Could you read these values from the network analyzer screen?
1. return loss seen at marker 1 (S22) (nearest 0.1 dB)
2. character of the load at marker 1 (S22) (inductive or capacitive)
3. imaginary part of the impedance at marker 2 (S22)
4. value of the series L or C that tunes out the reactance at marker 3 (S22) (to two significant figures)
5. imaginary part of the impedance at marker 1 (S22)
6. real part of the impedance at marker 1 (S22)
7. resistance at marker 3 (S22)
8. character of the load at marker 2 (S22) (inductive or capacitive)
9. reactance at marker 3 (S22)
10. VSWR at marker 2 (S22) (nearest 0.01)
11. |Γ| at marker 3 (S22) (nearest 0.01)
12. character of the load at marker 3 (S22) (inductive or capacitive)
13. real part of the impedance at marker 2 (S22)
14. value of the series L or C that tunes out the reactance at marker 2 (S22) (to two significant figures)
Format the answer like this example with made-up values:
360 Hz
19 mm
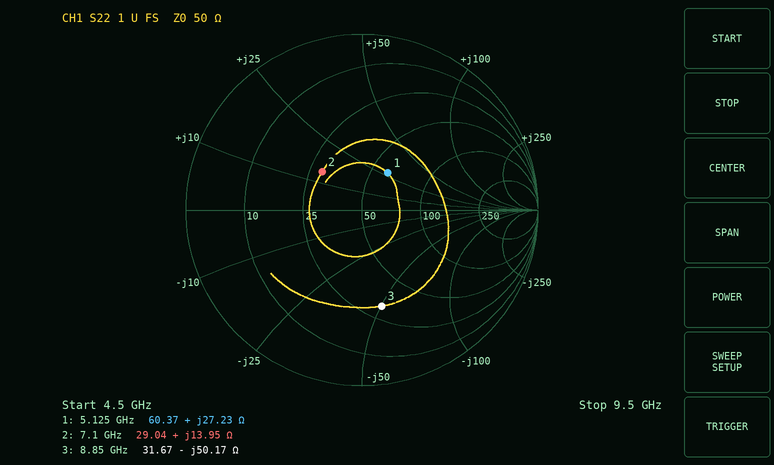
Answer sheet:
11.8 dB
inductive
+13.95 Ω
900 pH
+27.23 Ω
60.37 Ω
31.67 Ω
inductive
-50.17 Ω
1.91
0.56
capacitive
29.04 Ω
1.6 pF
